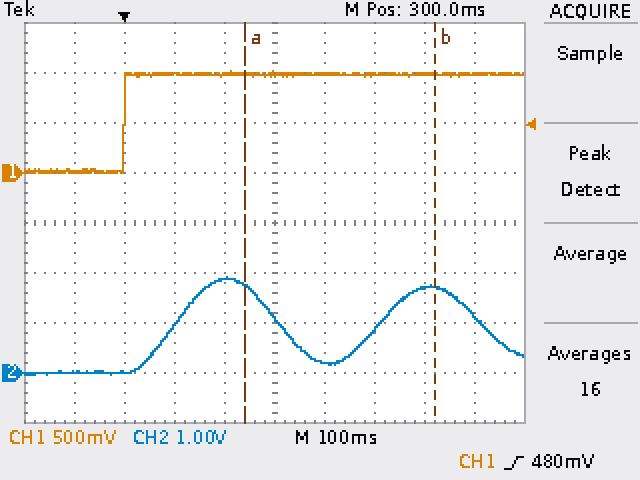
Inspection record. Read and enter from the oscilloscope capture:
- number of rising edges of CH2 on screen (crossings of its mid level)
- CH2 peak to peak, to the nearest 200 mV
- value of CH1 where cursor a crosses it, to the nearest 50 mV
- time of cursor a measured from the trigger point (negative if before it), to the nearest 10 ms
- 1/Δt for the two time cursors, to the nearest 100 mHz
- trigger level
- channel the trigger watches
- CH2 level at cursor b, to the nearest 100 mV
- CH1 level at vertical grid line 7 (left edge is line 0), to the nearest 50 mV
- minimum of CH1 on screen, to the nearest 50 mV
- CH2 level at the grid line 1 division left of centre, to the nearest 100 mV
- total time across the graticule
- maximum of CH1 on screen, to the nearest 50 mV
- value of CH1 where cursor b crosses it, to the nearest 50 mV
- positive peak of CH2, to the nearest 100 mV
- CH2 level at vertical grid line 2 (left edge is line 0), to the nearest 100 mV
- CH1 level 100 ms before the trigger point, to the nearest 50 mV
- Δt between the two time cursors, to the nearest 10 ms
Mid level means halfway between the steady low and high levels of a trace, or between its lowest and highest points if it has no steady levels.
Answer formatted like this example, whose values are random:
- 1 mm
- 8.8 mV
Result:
- 2
- 2.0 V
- 1.00 V
- +240 ms
- 2.6 Hz
- 480 mV
- CH1
- 1.7 V
- 1.00 V
- 0 mV
- 1.9 V
- 1 s
- 1.00 V
- 1.00 V
- 1.9 V
- 0.0 V
- 0 mV
- 380 ms
